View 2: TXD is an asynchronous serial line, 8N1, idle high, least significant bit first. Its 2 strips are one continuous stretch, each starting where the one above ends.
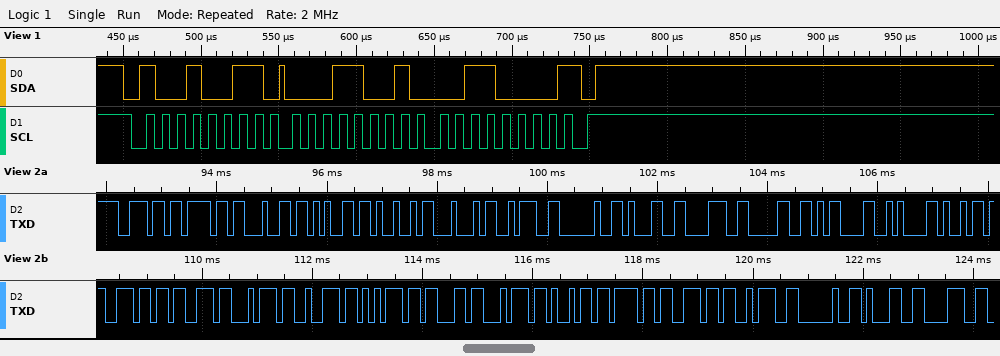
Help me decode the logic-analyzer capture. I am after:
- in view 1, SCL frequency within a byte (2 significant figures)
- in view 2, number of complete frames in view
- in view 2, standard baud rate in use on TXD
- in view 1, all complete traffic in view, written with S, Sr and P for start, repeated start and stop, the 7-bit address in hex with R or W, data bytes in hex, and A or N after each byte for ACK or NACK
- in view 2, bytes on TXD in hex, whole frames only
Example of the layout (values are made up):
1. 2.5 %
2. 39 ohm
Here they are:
1. 100 kHz
2. 28
3. 9600 baud
4. S 49R A 19 A 30 N P
5. 6E 6F 64 65 49 44 3A 20 31 38 30 0D 0A 69 6E 73 74 72 75 63 74 69 6F 6E 3A 20 31 38
